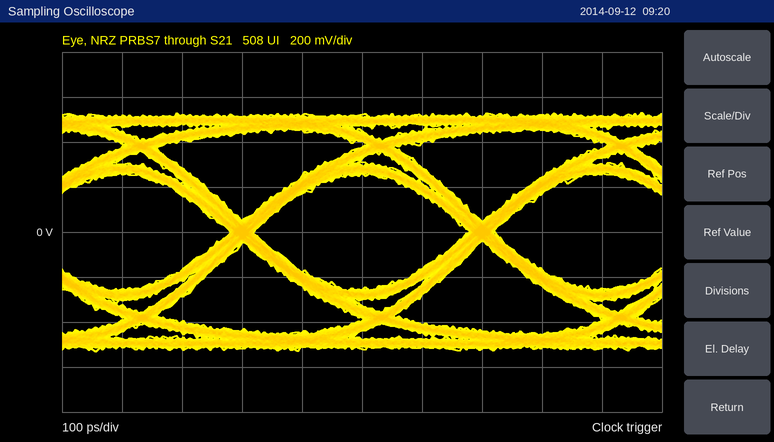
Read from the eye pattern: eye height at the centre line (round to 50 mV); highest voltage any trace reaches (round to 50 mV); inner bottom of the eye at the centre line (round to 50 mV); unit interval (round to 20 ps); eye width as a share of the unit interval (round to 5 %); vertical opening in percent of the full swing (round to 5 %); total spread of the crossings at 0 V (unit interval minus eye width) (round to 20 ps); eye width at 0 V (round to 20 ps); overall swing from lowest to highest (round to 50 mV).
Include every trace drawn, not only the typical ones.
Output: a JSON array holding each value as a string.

["500 mV", "550 mV", "-250 mV", "400 ps", "90 %", "50 %", "40 ps", "360 ps", "1.05 V"]
